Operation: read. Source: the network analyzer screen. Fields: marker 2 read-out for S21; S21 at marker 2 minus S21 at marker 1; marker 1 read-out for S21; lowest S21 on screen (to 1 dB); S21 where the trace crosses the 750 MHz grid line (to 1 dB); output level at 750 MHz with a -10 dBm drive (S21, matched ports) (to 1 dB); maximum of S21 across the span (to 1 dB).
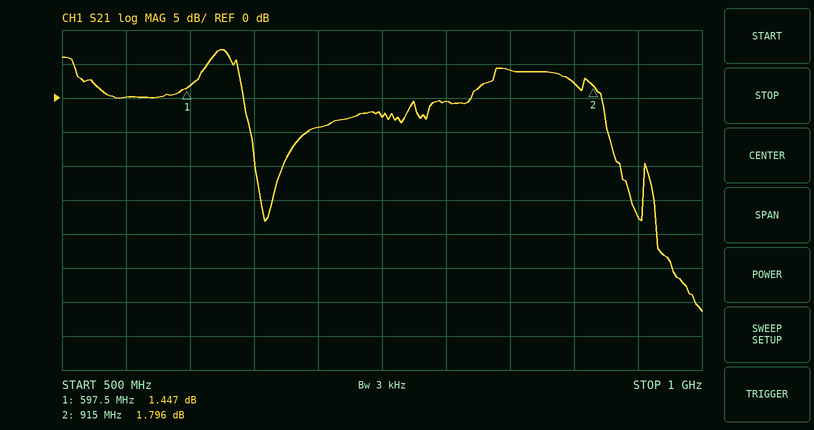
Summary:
1.796 dB
0.349 dB
1.447 dB
-31 dB
-3 dB
-13 dBm
7 dB
